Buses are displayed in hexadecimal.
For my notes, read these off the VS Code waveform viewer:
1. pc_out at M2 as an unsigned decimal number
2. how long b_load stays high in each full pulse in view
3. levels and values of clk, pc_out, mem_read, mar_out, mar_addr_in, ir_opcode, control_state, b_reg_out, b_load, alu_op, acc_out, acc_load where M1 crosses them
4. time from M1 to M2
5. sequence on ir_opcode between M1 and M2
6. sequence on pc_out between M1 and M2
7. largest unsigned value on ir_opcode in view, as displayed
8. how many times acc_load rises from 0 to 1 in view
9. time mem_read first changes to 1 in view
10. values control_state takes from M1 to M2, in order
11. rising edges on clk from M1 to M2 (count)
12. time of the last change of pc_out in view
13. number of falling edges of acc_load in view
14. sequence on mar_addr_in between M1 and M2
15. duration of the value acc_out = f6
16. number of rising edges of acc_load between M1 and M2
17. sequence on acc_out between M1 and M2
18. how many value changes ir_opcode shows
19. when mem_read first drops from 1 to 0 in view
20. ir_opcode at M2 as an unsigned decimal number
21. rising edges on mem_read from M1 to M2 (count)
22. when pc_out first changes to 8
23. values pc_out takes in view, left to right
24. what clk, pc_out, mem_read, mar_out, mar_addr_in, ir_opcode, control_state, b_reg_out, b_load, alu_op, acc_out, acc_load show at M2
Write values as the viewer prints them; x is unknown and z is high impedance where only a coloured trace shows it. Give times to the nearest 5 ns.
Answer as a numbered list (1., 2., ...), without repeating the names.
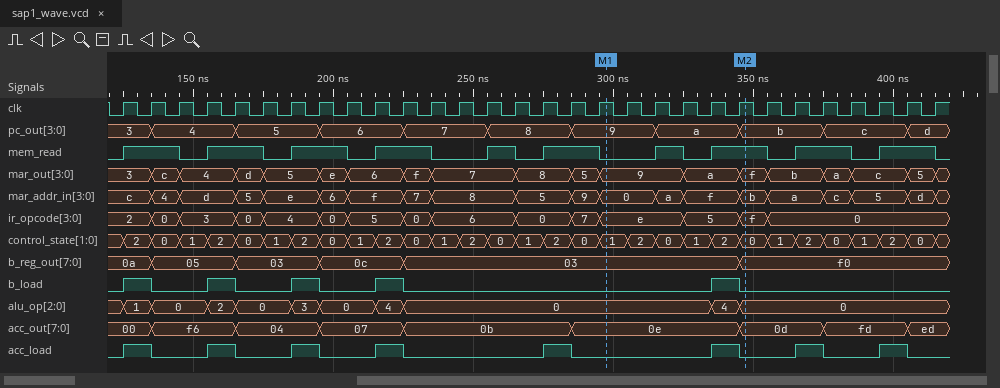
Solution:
1. 11
2. 10 ns, 10 ns, 10 ns, 10 ns, 10 ns
3. clk=1, pc_out=9, mem_read=0, mar_out=9, mar_addr_in=0, ir_opcode=e, control_state=1, b_reg_out=03, b_load=0, alu_op=0, acc_out=0e, acc_load=0
4. 50 ns
5. e, 5, f
6. 9, a, b
7. f
8. 8
9. 125 ns
10. 1, 2, 0, 1, 2, 0
11. 5
12. 405 ns
13. 8
14. 0, a, f, b
15. 30 ns
16. 1
17. 0e, 0d
18. 14
19. 145 ns
20. 15
21. 2
22. 255 ns
23. 3, 4, 5, 6, 7, 8, 9, a, b, c, d
24. clk=1, pc_out=b, mem_read=1, mar_out=f, mar_addr_in=b, ir_opcode=f, control_state=0, b_reg_out=f0, b_load=0, alu_op=0, acc_out=0d, acc_load=0
